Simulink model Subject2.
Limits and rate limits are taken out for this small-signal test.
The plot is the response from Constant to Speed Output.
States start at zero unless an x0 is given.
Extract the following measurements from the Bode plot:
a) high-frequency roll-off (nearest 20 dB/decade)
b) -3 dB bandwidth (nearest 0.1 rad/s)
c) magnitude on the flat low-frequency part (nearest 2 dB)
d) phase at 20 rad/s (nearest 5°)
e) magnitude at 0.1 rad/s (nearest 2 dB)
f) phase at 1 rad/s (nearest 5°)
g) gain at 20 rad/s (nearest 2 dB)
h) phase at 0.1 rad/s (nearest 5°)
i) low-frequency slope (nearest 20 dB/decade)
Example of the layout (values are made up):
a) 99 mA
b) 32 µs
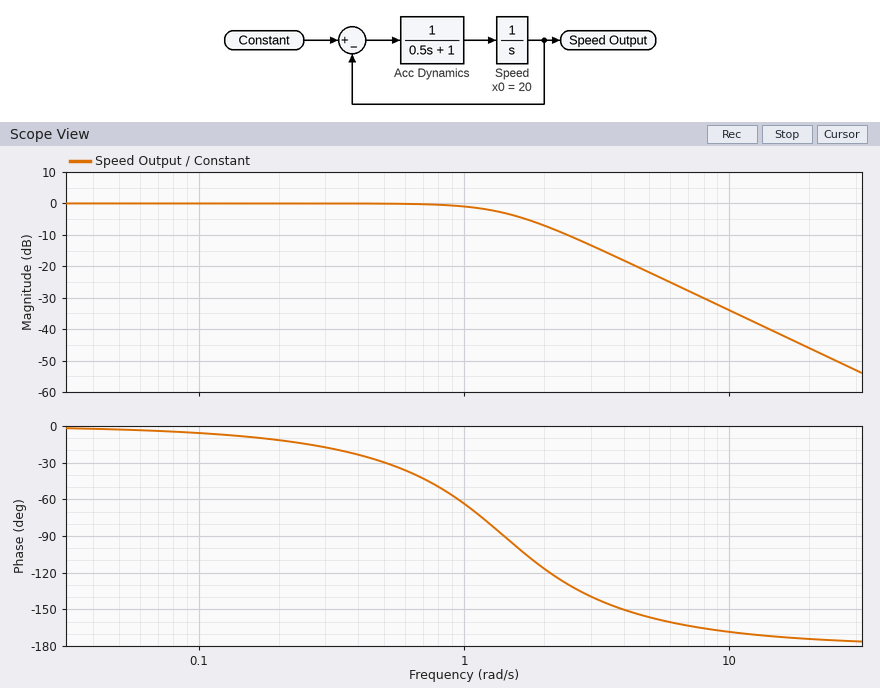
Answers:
a) -40 dB/decade
b) 1.4 rad/s
c) 0 dB
d) -175°
e) 0 dB
f) -65°
g) -46 dB
h) -5°
i) 0 dB/decade
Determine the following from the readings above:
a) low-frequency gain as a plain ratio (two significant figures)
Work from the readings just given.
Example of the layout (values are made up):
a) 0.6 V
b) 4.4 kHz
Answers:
a) 1.0
